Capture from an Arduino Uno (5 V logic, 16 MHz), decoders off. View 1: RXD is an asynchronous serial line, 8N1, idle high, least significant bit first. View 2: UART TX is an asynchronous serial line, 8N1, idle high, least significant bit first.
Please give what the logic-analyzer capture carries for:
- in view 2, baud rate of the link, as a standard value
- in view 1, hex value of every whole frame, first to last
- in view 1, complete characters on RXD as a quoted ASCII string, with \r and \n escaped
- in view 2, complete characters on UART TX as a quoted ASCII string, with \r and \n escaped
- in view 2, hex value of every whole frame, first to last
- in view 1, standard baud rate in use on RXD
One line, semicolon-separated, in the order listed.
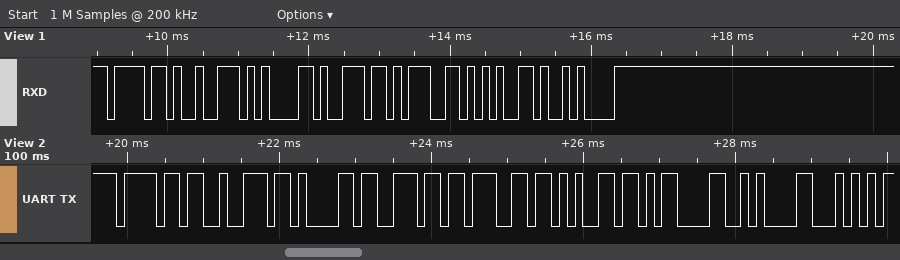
9600 baud; 0x6F 0x72 0x61 0x6E 0x67 0x65 0x0A; "orange\n"; "orange\r\nT"; 6F 72 61 6E 67 65 0D 0A 54; 9600 baud
